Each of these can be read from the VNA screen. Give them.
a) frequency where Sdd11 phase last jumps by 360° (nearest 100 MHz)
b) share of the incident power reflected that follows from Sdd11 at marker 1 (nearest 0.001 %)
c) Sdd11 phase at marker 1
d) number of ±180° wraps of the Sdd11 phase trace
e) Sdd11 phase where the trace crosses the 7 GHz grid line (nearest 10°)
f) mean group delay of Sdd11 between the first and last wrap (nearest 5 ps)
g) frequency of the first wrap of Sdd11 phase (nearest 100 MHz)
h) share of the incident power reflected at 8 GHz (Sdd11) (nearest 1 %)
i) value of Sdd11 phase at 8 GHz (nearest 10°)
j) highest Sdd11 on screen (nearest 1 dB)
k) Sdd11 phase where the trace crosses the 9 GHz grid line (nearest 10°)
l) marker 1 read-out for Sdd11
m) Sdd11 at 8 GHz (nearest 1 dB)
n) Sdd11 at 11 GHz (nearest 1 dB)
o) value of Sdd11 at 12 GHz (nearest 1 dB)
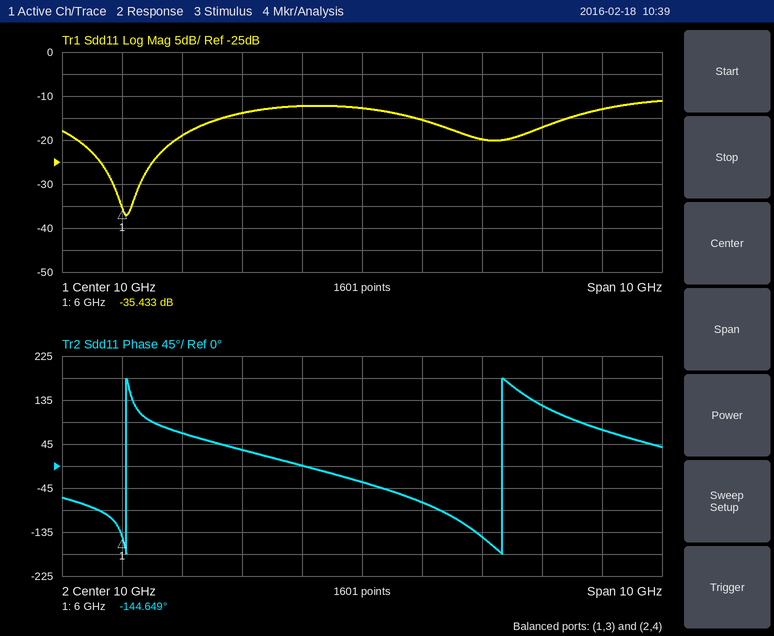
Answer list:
12.3 GHz
0.029 %
-144.649°
2
70°
160 ps
6.1 GHz
4 %
30°
-11 dB
0°
-35.433 dB
-14 dB
-15 dB
-20 dB
